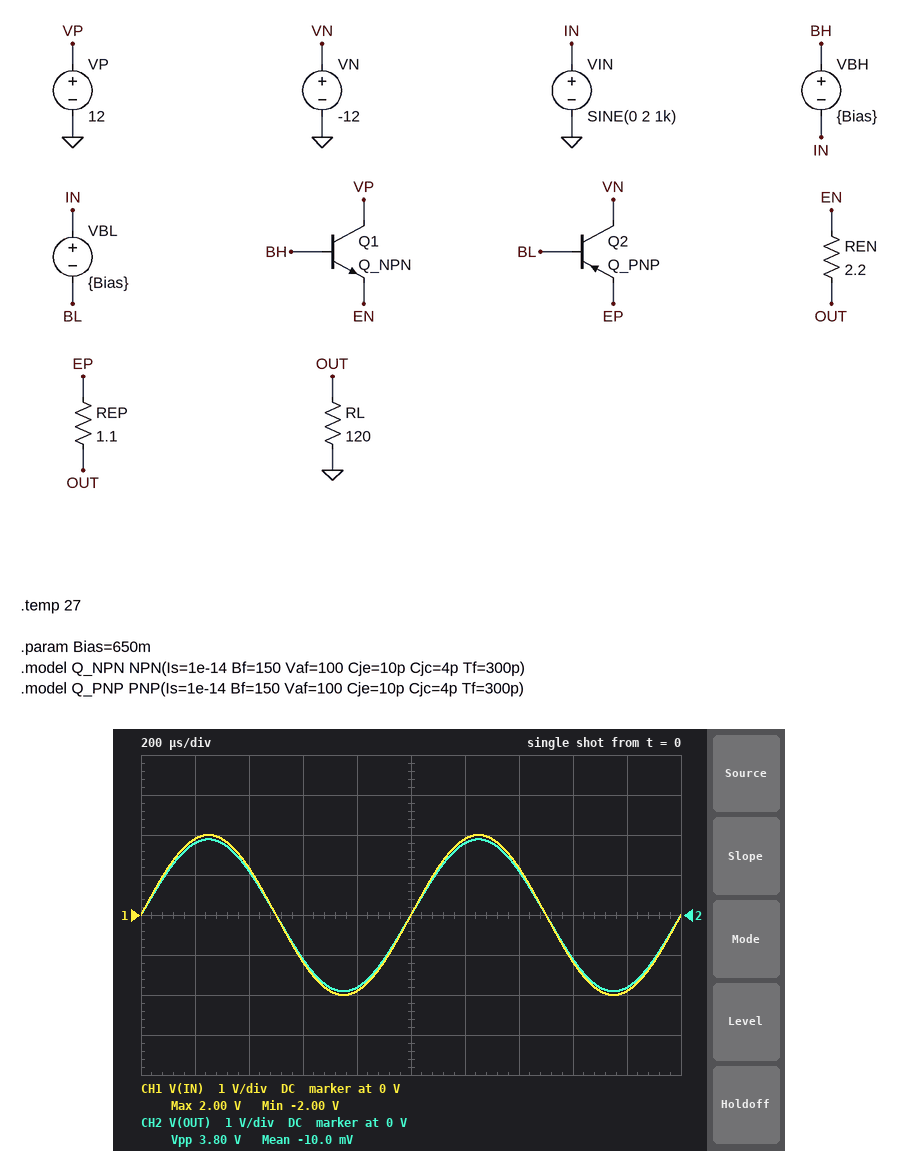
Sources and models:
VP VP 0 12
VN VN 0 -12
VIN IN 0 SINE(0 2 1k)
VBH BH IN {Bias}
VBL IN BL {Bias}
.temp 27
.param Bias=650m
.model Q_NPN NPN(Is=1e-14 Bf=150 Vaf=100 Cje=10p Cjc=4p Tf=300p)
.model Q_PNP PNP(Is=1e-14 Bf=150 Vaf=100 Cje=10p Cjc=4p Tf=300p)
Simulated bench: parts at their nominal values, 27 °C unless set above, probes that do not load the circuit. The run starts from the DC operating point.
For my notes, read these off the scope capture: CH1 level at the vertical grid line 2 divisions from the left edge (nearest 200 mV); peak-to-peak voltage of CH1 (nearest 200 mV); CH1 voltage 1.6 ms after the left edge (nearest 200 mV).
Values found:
1.2 V
4.0 V
-1.2 V
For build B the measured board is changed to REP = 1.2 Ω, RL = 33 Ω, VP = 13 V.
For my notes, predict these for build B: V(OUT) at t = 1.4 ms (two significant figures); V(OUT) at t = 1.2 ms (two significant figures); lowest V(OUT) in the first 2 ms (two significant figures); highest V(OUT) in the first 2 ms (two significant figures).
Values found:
1.0 V
1.7 V
-1.8 V
1.8 V
